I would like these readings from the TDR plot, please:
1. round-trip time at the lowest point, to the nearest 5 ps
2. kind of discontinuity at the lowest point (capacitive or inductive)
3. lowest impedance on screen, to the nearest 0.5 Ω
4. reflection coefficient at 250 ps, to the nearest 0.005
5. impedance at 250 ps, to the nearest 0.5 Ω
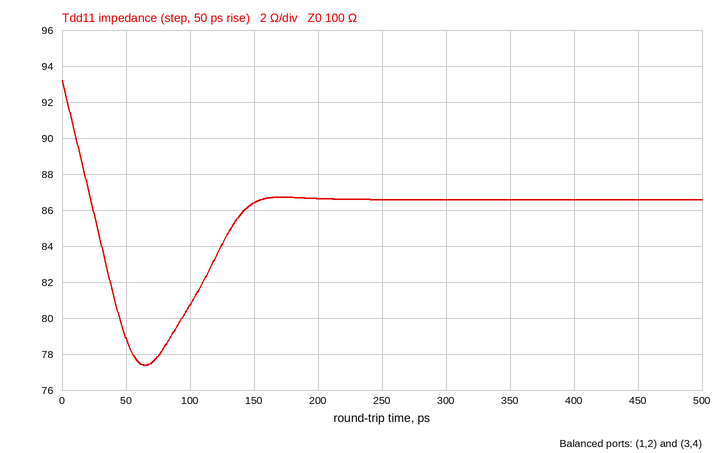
65 ps
capacitive
77.5 Ω
-0.070
86.5 Ω
